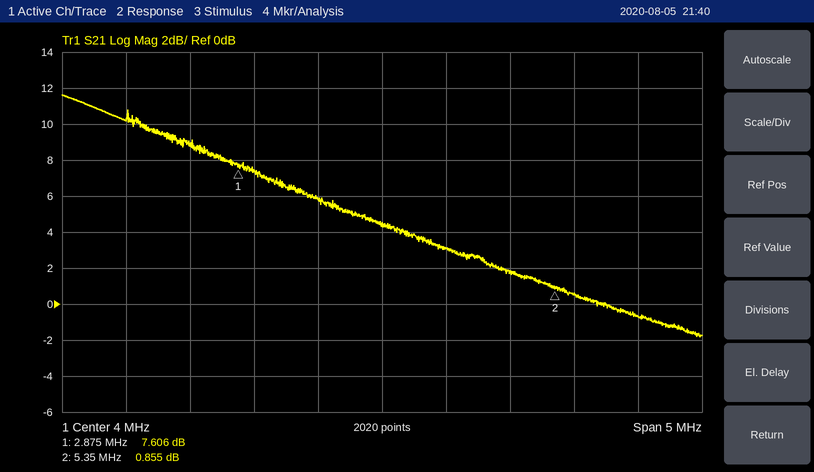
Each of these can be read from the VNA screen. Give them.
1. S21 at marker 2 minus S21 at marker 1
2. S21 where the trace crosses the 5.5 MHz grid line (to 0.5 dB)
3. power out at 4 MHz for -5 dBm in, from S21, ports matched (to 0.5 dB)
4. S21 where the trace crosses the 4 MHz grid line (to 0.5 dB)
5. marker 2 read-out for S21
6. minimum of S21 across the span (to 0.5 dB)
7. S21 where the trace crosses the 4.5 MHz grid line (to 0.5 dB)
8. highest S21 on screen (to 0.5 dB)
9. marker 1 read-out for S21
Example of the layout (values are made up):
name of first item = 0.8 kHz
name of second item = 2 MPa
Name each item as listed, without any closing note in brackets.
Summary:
S21 at marker 2 minus S21 at marker 1 = -6.751 dB
S21 where the trace crosses the 5.5 MHz grid line = 0.5 dB
power out at 4 MHz for -5 dBm in, from S21, ports matched = -0.5 dBm
S21 where the trace crosses the 4 MHz grid line = 4.5 dB
marker 2 read-out for S21 = 0.855 dB
minimum of S21 across the span = -2.0 dB
S21 where the trace crosses the 4.5 MHz grid line = 3.0 dB
highest S21 on screen = 11.5 dB
marker 1 read-out for S21 = 7.606 dB
